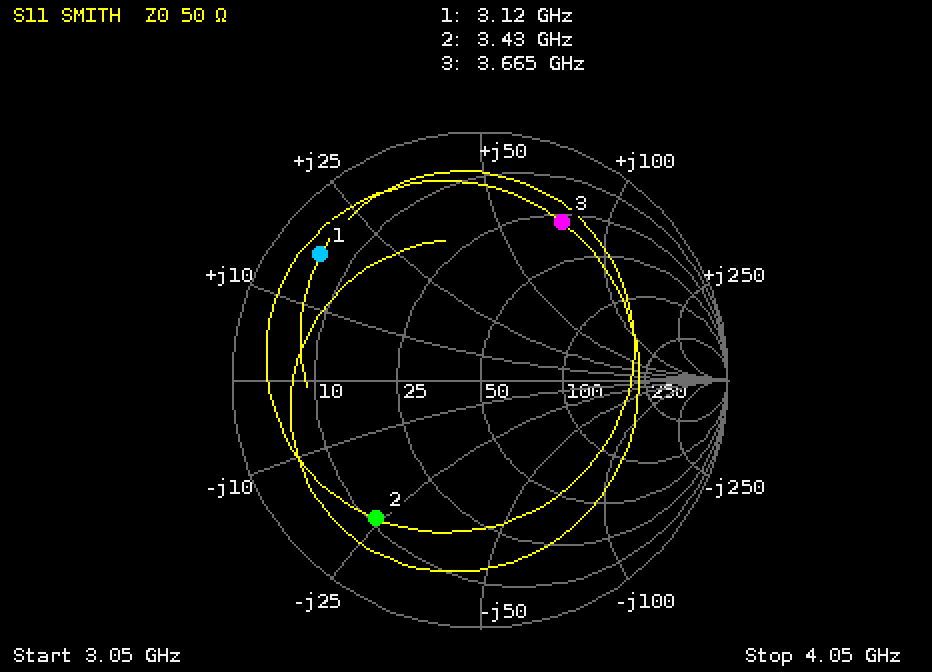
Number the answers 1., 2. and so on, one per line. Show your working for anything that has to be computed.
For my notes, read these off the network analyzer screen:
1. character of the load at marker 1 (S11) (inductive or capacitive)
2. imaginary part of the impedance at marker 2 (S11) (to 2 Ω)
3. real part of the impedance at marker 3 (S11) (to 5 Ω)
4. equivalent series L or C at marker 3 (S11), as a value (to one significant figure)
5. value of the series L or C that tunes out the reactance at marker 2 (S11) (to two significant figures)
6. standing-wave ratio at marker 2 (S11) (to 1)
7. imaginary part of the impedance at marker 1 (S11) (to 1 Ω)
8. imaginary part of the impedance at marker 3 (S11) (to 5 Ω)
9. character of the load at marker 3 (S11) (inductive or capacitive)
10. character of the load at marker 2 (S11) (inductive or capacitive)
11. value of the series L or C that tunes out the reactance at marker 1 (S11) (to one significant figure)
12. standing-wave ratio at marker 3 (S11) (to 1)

1. inductive
2. -24 Ω
3. 30 Ω
4. L = 75 Ω/(2π × 3.665 GHz) ≈ 3 nH
5. L = 24 Ω/(2π × 3.43 GHz) ≈ 1.1 nH
6. 6
7. +17 Ω
8. +75 Ω
9. inductive
10. capacitive
11. C = 1/(2π × 3.12 GHz × 17 Ω) ≈ 3 pF
12. 6
